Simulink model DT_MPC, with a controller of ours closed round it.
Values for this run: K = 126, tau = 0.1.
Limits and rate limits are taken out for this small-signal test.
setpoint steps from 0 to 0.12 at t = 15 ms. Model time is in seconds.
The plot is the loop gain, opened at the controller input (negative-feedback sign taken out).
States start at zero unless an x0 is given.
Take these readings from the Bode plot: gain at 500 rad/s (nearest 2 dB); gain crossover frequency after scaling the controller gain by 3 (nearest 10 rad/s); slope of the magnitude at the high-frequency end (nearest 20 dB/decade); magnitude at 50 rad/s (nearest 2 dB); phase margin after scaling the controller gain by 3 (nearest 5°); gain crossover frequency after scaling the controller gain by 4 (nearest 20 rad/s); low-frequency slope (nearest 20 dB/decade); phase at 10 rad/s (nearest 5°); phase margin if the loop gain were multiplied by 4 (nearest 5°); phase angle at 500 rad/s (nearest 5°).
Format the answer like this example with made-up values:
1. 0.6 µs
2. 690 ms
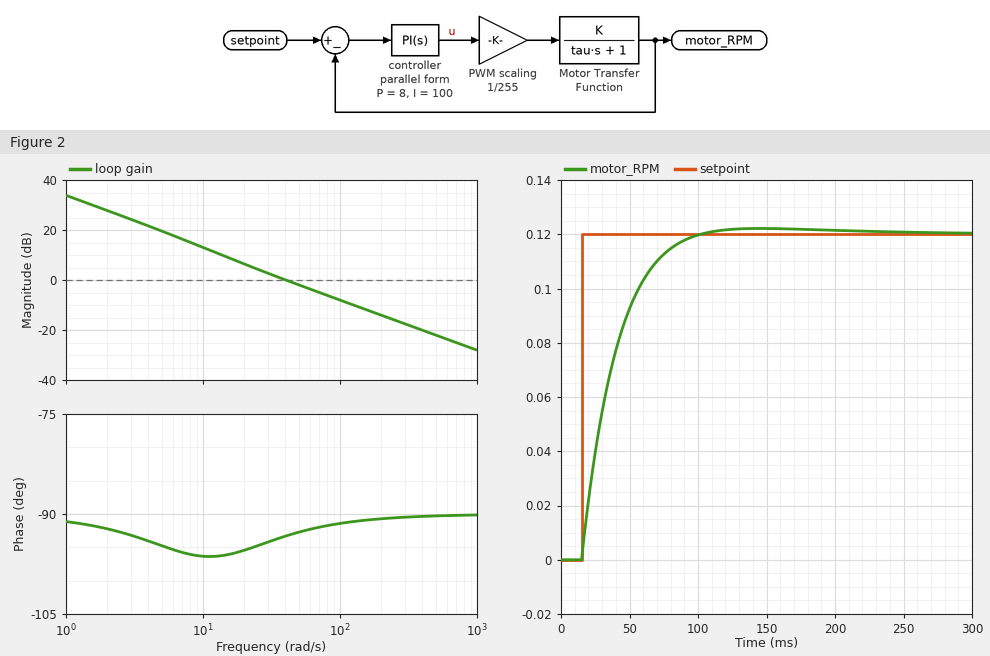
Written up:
1. -22 dB
2. 120 rad/s
3. -20 dB/decade
4. -2 dB
5. 90°
6. 160 rad/s
7. -20 dB/decade
8. -95°
9. 90°
10. -90°
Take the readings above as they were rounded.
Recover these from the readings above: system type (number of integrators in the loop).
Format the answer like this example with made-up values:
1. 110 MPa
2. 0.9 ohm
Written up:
1. 1
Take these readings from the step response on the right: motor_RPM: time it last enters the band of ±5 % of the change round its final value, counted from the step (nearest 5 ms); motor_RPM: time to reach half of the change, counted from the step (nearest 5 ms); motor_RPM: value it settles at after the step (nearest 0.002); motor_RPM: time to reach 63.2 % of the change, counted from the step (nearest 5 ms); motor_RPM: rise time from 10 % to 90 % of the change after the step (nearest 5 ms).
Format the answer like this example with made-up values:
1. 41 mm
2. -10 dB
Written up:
1. 65 ms
2. 15 ms
3. 0.120
4. 25 ms
5. 50 ms
